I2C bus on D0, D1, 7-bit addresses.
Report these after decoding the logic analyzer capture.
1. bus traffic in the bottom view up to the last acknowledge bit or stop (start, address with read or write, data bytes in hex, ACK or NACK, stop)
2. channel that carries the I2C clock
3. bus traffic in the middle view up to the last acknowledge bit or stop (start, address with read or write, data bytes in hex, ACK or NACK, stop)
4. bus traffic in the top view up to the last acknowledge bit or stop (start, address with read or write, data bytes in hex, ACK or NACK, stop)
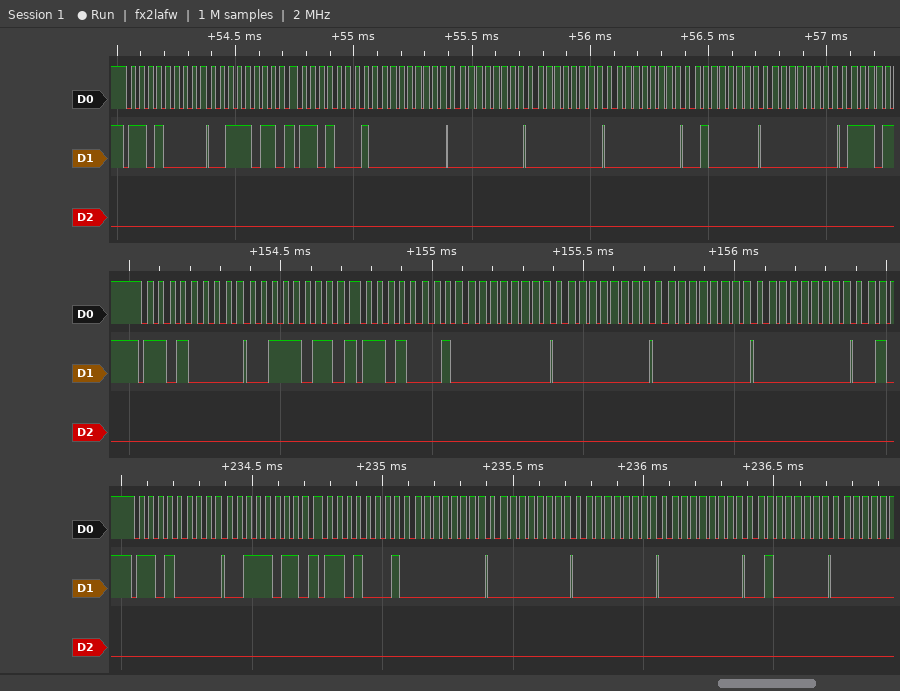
start, address 68 write ACK, 3B ACK, repeated start, address 68 read ACK, 00 ACK, 00 ACK, 00 ACK, 00 ACK, 40 ACK
D0
start, address 68 write ACK, 3B ACK, repeated start, address 68 read ACK, 00 ACK, 00 ACK, 00 ACK, 00 ACK
start, address 68 write ACK, 3B ACK, repeated start, address 68 read ACK, 00 ACK, 00 ACK, 00 ACK, 00 ACK, 40 ACK, 00 ACK
